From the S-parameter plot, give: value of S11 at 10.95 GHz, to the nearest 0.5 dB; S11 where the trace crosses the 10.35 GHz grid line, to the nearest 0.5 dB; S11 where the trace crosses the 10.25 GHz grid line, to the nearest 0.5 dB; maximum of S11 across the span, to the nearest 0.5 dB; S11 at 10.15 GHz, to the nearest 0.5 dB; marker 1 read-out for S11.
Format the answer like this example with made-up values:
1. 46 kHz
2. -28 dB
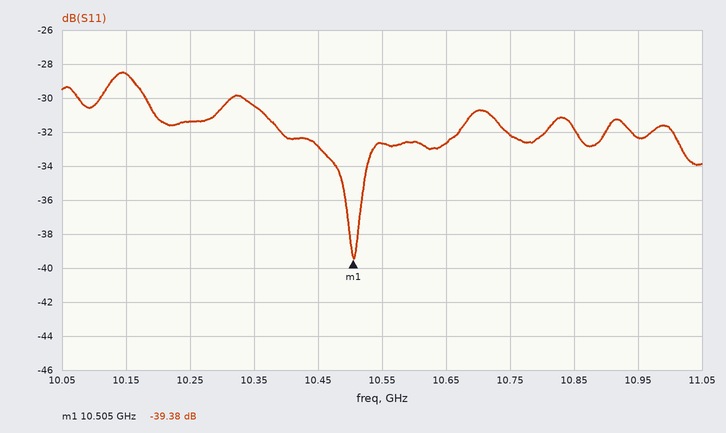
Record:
1. -32.5 dB
2. -30.5 dB
3. -31.5 dB
4. -28.5 dB
5. -28.5 dB
6. -39.38 dB
